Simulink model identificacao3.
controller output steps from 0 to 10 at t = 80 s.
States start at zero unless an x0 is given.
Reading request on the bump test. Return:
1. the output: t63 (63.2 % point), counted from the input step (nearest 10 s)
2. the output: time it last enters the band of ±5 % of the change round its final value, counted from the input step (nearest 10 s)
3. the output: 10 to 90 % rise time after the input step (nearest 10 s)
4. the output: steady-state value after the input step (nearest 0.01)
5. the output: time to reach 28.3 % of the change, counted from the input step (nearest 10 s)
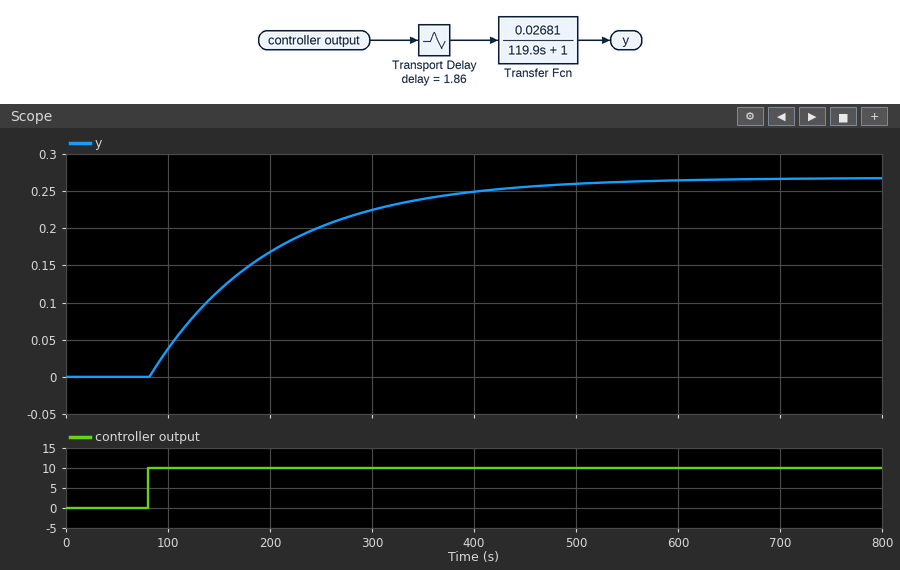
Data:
120 s
360 s
260 s
0.27
40 s
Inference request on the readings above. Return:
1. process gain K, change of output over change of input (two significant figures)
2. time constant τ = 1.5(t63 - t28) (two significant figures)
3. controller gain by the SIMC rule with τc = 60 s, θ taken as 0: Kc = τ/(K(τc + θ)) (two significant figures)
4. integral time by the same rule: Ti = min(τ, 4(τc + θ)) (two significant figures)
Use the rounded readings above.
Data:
0.027
120 s
74
120 s
